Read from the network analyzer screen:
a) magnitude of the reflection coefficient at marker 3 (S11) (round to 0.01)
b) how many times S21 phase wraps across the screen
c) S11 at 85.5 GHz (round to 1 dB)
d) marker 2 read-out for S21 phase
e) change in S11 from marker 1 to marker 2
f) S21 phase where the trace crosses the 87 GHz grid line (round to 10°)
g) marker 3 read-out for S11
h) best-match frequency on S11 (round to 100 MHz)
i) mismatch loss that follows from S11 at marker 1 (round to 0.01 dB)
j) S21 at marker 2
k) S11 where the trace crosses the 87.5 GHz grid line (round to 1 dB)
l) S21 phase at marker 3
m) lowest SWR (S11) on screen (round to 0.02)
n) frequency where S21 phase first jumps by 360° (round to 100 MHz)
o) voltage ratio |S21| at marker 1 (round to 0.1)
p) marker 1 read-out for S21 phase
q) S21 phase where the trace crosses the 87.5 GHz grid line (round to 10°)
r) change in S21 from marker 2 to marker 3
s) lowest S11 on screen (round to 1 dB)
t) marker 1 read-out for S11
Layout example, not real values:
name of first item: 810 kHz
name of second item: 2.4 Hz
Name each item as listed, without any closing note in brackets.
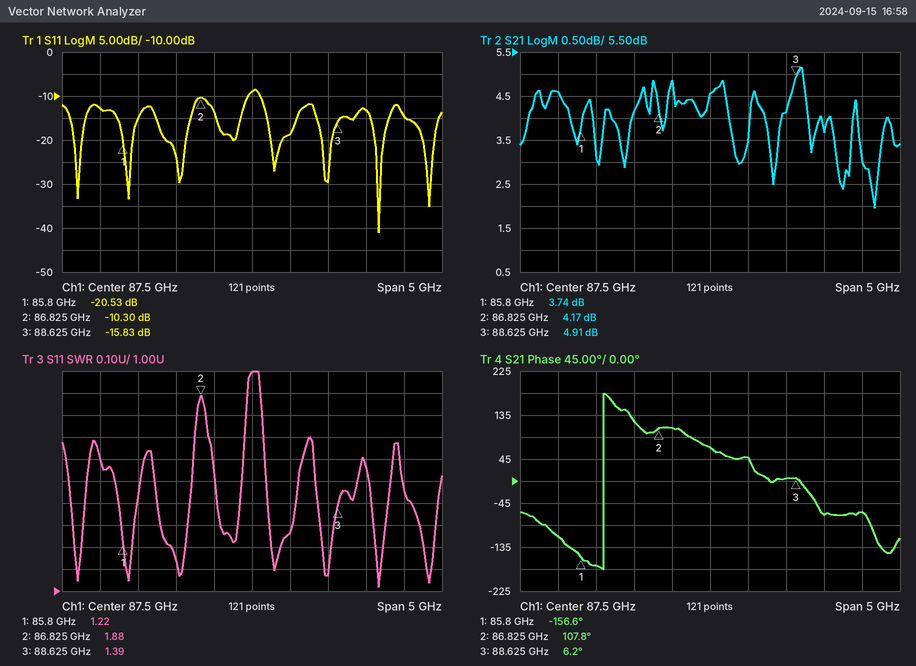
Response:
magnitude of the reflection coefficient at marker 3 (S11): 0.16
how many times S21 phase wraps across the screen: 1
S11 at 85.5 GHz: -13 dB
marker 2 read-out for S21 phase: 107.8°
change in S11 from marker 1 to marker 2: 10.23 dB
S21 phase where the trace crosses the 87 GHz grid line: 110°
marker 3 read-out for S11: -15.83 dB
best-match frequency on S11: 89.2 GHz
mismatch loss that follows from S11 at marker 1: 0.04 dB
S21 at marker 2: 4.17 dB
S11 where the trace crosses the 87.5 GHz grid line: -9 dB
S21 phase at marker 3: 6.2°
lowest SWR (S11) on screen: 1.02
frequency where S21 phase first jumps by 360°: 86.1 GHz
voltage ratio |S21| at marker 1: 1.5
marker 1 read-out for S21 phase: -156.6°
S21 phase where the trace crosses the 87.5 GHz grid line: 70°
change in S21 from marker 2 to marker 3: 0.74 dB
lowest S11 on screen: -41 dB
marker 1 read-out for S11: -20.53 dB
